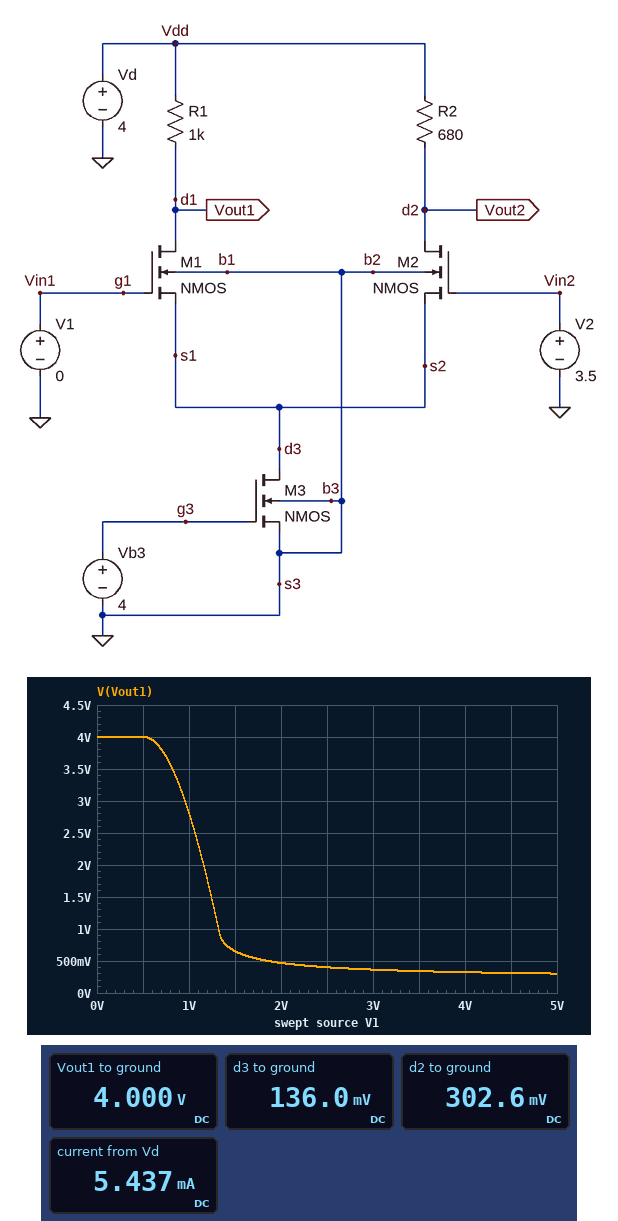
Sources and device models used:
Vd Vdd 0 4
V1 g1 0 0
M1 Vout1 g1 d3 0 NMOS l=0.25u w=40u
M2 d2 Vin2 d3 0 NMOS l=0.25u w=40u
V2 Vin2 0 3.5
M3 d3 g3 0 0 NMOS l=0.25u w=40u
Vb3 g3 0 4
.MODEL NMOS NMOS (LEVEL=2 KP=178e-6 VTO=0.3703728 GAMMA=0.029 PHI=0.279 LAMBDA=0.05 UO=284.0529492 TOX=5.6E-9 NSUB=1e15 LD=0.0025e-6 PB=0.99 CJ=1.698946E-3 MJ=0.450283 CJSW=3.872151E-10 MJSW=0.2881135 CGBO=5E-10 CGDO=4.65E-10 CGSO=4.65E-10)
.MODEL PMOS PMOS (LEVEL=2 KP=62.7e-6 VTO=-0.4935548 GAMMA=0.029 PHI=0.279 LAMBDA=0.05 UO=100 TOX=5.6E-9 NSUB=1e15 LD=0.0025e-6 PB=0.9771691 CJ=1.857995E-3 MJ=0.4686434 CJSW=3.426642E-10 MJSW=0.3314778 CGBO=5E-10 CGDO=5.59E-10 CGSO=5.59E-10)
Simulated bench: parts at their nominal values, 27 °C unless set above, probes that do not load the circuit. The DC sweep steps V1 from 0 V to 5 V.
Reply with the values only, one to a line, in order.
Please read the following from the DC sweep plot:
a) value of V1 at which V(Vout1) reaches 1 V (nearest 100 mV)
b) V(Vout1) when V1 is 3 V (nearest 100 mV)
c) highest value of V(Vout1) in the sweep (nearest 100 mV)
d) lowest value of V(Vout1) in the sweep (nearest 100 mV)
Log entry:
1.3 V
400 mV
4.0 V
300 mV
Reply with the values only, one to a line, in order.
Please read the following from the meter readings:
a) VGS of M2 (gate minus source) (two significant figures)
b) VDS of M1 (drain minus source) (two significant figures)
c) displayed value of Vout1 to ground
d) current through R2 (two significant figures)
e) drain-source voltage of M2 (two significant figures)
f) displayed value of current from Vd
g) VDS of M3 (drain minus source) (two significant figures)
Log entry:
3.4 V
3.9 V
4.000 V
5.4 mA
170 mV
5.437 mA
140 mV
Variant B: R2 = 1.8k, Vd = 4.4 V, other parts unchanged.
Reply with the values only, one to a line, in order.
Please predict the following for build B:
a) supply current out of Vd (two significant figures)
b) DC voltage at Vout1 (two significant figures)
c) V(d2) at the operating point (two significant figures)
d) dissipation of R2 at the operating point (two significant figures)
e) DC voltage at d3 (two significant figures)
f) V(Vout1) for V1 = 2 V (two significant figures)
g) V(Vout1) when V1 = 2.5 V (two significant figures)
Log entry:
2.4 mA
4.4 V
130 mV
10 mW
59 mV
420 mV
350 mV
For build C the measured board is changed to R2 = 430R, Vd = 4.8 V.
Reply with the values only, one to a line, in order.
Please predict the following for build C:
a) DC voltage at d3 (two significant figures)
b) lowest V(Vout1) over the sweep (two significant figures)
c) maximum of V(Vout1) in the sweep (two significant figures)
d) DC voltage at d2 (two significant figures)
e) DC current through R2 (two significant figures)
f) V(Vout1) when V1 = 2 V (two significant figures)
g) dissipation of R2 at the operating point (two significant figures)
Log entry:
250 mV
450 mV
4.8 V
570 mV
9.8 mA
690 mV
42 mW
